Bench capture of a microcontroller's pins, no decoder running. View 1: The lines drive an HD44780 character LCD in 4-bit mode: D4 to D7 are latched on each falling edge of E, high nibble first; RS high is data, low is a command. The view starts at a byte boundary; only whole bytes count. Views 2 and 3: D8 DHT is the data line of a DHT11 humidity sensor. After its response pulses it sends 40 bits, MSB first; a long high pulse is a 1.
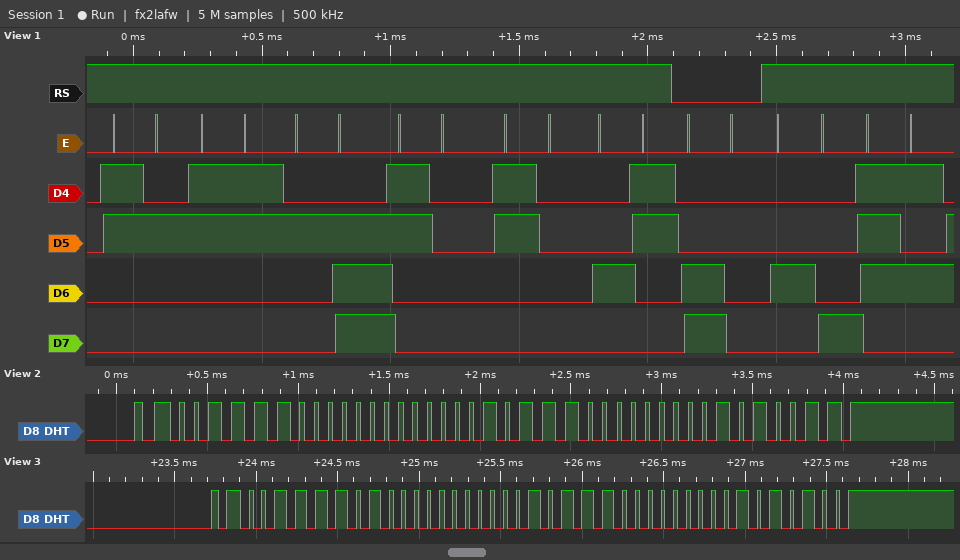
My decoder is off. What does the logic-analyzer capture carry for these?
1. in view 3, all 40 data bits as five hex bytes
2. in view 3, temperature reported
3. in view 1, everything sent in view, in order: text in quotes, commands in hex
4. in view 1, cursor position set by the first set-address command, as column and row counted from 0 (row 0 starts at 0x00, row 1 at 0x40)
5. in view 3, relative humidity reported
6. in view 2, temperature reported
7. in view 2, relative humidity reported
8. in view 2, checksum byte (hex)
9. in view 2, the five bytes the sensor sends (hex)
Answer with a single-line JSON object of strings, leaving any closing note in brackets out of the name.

{"in view 3, all 40 data bits as five hex bytes": "3D 00 17 00 54", "in view 3, temperature reported": "23.0 °C", "in view 1, everything sent in view, in order: text in quotes, commands in hex": "\"23.00C\" 0xC0 \"Hu\"", "in view 1, cursor position set by the first set-address command, as column and row counted from 0": "column 0, row 1", "in view 3, relative humidity reported": "61 %", "in view 2, temperature reported": "23.0 °C", "in view 2, relative humidity reported": "60 %", "in view 2, checksum byte": "0x53", "in view 2, the five bytes the sensor sends": "3C 00 17 00 53"}
